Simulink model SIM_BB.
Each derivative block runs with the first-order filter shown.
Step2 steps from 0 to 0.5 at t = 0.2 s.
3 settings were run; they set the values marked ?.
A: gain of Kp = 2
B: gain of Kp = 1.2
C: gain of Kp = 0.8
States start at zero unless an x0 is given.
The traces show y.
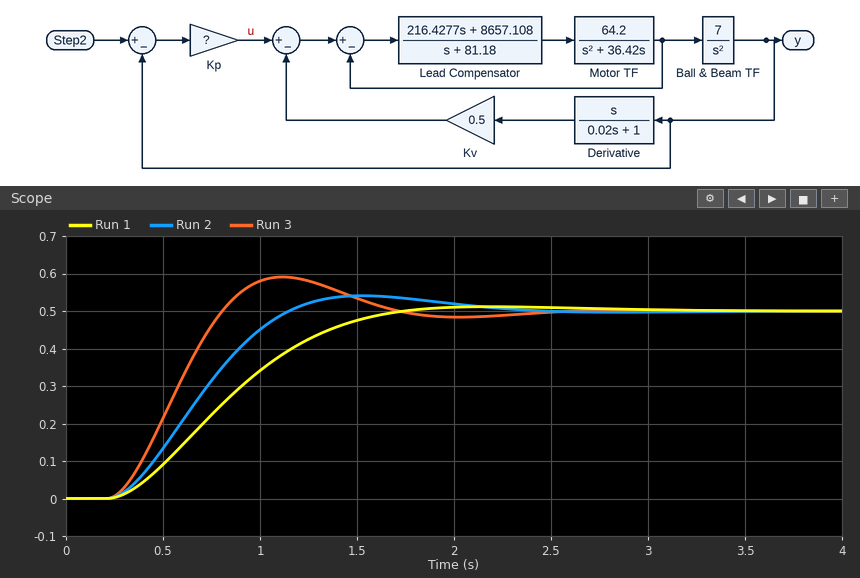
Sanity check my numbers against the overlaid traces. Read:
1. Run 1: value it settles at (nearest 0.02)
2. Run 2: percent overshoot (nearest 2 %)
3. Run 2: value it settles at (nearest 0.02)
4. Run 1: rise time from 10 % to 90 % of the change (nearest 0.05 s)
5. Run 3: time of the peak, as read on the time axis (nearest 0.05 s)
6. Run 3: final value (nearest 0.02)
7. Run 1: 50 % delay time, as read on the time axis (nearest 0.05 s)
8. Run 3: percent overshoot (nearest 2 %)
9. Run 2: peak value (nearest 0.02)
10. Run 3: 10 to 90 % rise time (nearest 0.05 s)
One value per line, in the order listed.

0.50
8 %
0.50
0.95 s
1.10 s
0.50
0.80 s
18 %
0.54
0.40 s
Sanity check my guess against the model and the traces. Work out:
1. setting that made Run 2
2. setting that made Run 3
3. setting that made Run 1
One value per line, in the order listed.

B
A
C
